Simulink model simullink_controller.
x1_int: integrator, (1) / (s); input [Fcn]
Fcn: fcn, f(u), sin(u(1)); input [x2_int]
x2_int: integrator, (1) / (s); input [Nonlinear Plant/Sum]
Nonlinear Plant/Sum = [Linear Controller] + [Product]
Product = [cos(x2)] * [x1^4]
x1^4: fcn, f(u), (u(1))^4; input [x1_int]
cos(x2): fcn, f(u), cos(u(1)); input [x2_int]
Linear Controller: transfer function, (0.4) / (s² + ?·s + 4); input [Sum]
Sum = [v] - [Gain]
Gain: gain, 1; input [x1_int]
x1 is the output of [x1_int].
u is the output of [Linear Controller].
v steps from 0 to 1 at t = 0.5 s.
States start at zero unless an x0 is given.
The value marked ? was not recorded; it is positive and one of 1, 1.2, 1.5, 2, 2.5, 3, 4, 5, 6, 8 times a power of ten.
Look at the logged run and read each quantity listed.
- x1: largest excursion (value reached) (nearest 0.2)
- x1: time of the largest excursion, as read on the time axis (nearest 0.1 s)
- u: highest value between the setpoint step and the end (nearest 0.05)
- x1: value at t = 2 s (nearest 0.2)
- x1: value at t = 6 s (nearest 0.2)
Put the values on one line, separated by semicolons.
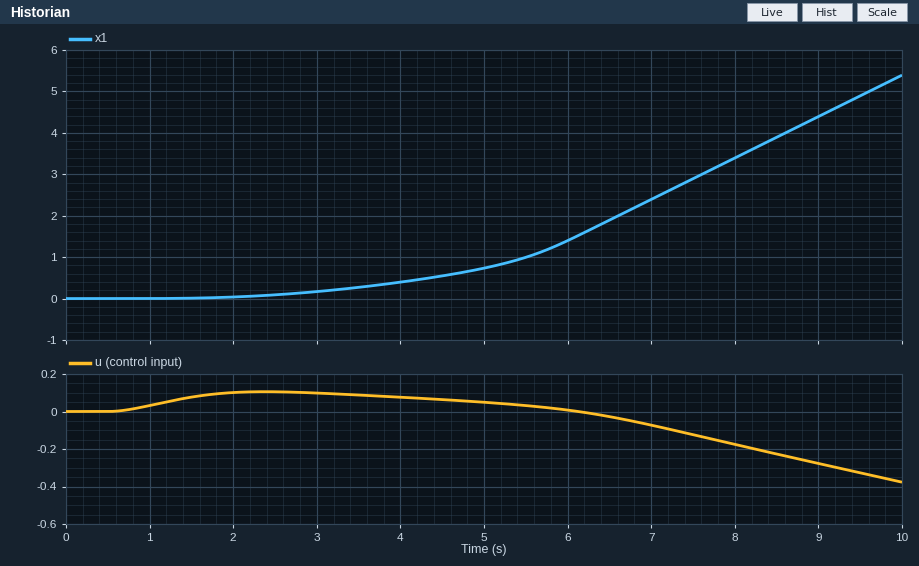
5.4; 10.0 s; 0.10; 0.0; 1.4
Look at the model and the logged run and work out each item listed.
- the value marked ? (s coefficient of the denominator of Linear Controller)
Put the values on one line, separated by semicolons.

2.5
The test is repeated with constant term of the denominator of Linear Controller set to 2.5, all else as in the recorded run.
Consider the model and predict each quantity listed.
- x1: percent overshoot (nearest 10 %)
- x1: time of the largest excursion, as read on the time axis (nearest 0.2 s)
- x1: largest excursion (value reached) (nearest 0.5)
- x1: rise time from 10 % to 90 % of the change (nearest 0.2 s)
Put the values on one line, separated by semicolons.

70 %; 10.0 s; 6.0; 3.6 s
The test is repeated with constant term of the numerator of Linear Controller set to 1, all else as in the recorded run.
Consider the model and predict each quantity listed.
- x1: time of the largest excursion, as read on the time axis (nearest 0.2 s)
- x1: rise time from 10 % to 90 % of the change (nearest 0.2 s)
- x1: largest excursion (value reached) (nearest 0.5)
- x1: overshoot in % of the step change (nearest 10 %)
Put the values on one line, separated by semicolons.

10.0 s; 3.4 s; 7.0; 100 %
